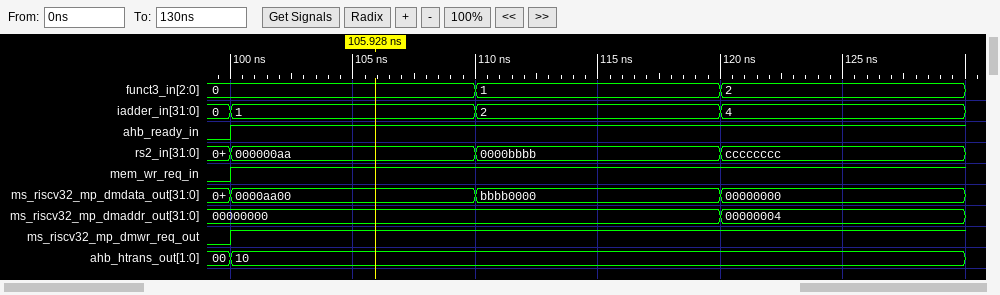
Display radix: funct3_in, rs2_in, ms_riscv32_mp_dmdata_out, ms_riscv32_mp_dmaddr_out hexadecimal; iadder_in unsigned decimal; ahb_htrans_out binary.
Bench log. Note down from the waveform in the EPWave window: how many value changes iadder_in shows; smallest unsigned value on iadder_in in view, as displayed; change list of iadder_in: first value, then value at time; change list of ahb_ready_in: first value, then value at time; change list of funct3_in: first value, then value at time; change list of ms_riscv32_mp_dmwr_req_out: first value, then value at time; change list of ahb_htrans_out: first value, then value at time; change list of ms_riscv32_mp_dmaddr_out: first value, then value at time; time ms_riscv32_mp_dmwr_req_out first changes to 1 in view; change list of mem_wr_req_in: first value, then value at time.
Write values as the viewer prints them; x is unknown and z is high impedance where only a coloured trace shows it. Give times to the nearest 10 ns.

3
0
0, 1 at 100 ns, 2 at 110 ns, 4 at 120 ns
0, 1 at 100 ns
0, 1 at 110 ns, 2 at 120 ns
0, 1 at 100 ns
00, 10 at 100 ns
00000000, 00000004 at 120 ns
100 ns
0, 1 at 100 ns
